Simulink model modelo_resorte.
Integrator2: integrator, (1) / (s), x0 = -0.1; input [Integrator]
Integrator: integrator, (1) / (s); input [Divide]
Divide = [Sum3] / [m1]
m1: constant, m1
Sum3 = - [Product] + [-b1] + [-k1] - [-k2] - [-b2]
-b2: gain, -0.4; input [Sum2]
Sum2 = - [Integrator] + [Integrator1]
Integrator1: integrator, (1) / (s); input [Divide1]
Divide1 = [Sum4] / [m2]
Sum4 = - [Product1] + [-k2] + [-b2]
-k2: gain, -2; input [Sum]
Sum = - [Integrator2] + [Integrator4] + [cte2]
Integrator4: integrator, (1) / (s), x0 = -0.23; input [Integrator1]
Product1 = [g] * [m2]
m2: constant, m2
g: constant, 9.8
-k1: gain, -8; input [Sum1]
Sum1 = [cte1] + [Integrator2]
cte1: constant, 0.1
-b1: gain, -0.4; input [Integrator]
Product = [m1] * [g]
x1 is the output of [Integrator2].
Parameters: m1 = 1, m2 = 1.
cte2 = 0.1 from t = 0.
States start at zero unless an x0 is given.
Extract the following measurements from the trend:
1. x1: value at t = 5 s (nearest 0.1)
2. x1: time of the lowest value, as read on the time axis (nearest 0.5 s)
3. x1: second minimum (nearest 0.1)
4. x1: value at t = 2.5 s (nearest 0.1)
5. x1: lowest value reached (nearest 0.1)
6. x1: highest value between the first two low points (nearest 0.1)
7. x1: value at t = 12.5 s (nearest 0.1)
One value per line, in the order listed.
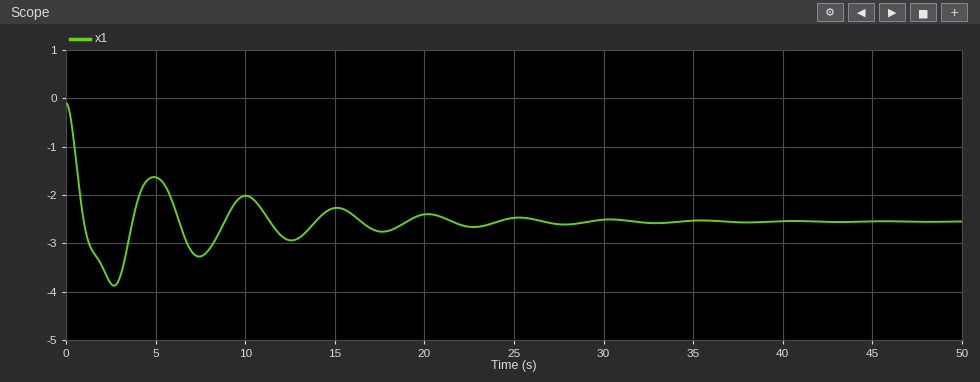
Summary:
-1.6
2.5 s
-3.3
-3.8
-3.9
-1.6
-2.9
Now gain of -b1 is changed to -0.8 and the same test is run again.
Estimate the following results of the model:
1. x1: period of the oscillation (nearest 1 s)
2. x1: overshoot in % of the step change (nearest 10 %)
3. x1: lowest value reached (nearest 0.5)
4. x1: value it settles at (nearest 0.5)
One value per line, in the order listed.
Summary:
5 s
50 %
-4.0
-2.5
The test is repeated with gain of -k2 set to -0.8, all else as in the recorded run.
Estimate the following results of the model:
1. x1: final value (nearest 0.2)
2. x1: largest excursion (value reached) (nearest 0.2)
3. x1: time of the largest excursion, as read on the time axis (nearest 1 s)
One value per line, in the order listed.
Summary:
-2.6
-3.6
3 s
